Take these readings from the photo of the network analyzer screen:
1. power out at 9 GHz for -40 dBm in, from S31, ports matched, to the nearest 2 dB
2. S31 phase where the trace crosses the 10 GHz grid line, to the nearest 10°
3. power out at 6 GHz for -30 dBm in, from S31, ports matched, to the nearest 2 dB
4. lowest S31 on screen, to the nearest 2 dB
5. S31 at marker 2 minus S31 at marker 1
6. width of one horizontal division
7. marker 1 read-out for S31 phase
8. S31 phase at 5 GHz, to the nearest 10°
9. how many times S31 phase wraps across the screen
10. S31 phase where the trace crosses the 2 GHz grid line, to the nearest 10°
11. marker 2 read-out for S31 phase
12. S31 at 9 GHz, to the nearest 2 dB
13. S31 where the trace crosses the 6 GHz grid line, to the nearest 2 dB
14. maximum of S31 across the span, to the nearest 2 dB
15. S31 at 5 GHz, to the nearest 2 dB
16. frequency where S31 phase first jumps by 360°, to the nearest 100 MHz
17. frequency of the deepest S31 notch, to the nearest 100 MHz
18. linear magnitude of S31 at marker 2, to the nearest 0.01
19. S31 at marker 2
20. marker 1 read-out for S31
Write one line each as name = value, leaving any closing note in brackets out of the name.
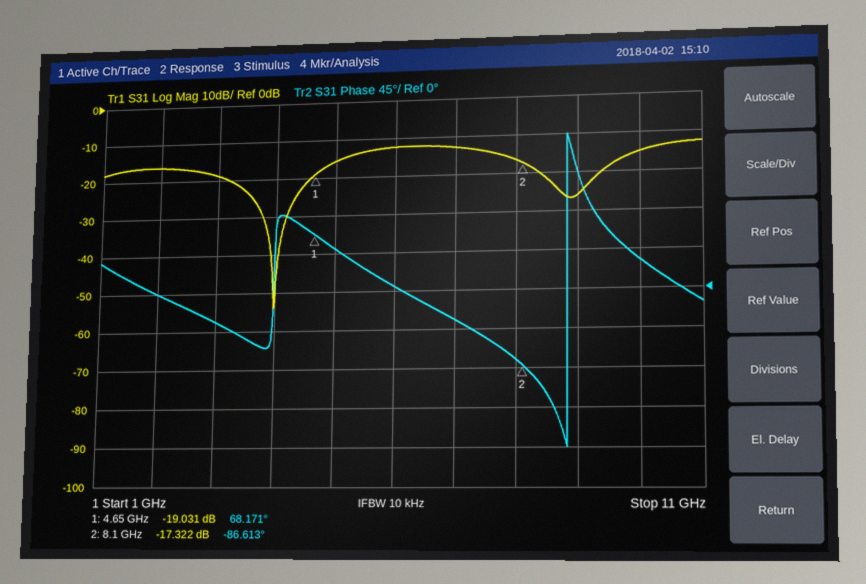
power out at 9 GHz for -40 dBm in, from S31, ports matched, to the nearest 2 dB = -66 dBm
S31 phase where the trace crosses the 10 GHz grid line, to the nearest 10° = 30°
power out at 6 GHz for -30 dBm in, from S31, ports matched, to the nearest 2 dB = -42 dBm
lowest S31 on screen, to the nearest 2 dB = -54 dB
S31 at marker 2 minus S31 at marker 1 = 1.709 dB
width of one horizontal division = 1 GHz
marker 1 read-out for S31 phase = 68.171°
S31 phase at 5 GHz, to the nearest 10° = 50°
how many times S31 phase wraps across the screen = 1
S31 phase where the trace crosses the 2 GHz grid line, to the nearest 10° = 0°
marker 2 read-out for S31 phase = -86.613°
S31 at 9 GHz, to the nearest 2 dB = -26 dB
S31 where the trace crosses the 6 GHz grid line, to the nearest 2 dB = -12 dB
maximum of S31 across the span, to the nearest 2 dB = -12 dB
S31 at 5 GHz, to the nearest 2 dB = -16 dB
frequency where S31 phase first jumps by 360°, to the nearest 100 MHz = 8.8 GHz
frequency of the deepest S31 notch, to the nearest 100 MHz = 4.0 GHz
linear magnitude of S31 at marker 2, to the nearest 0.01 = 0.14
S31 at marker 2 = -17.322 dB
marker 1 read-out for S31 = -19.031 dB
